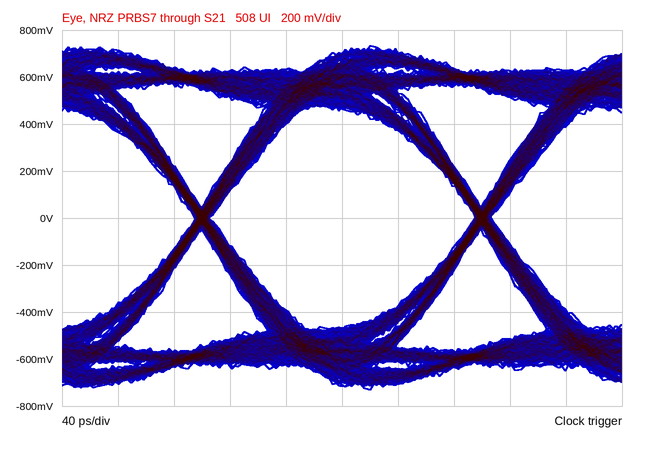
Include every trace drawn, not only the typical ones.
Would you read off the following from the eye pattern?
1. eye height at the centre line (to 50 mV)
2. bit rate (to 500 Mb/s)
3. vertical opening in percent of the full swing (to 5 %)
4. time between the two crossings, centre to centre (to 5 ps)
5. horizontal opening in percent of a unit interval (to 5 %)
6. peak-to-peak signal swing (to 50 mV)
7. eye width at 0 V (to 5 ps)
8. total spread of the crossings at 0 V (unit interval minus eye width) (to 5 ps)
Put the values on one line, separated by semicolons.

950 mV; 5.0 Gb/s; 65 %; 200 ps; 95 %; 1.45 V; 190 ps; 10 ps
